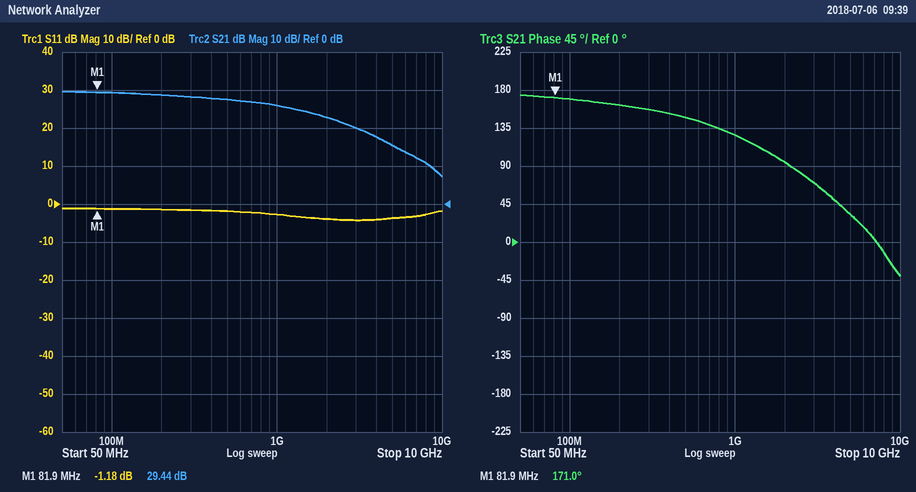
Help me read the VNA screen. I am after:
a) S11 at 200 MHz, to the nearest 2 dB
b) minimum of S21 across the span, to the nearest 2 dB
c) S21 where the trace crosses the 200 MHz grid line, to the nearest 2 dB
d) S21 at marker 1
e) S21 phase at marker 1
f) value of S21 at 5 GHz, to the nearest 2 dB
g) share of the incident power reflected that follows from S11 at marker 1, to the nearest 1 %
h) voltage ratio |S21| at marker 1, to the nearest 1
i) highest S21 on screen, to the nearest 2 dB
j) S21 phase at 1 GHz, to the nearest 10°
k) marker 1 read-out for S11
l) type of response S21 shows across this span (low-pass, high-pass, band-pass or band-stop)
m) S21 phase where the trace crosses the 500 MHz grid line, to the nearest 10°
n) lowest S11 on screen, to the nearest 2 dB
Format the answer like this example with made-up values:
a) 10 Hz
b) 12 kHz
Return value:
a) -2 dB
b) 8 dB
c) 28 dB
d) 29.44 dB
e) 171.0°
f) 16 dB
g) 76 %
h) 30
i) 30 dB
j) 130°
k) -1.18 dB
l) low-pass
m) 150°
n) -4 dB
